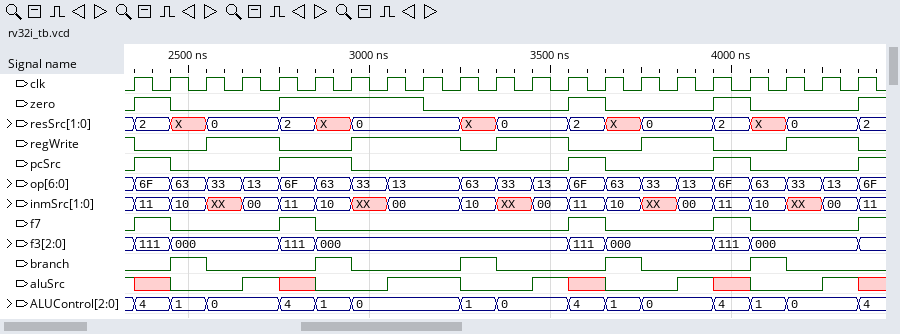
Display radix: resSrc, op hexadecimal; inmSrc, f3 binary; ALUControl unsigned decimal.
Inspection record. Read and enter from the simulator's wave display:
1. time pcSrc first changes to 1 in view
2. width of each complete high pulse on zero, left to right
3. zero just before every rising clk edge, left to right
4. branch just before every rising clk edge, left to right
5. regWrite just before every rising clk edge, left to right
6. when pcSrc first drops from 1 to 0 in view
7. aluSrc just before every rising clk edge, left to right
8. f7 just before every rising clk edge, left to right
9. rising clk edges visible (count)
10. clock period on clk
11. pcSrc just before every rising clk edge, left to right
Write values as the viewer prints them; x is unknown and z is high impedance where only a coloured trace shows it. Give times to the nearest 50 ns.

2350 ns
100 ns, 400 ns, 100 ns, 100 ns
0 1 0 0 0 1 1 1 1 0 0 0 0 1 0 0 0 1 0 0 0
0 0 1 0 0 0 1 0 0 0 1 0 0 0 1 0 0 0 1 0 0
1 0 0 1 1 0 0 1 1 1 0 1 1 0 0 1 1 0 0 1 1
2450 ns
1 x 0 0 1 x 0 0 1 1 0 0 1 x 0 0 1 x 0 0 1
0 1 0 0 0 1 0 0 0 0 0 0 0 1 0 0 0 1 0 0 0
21
100 ns
0 1 0 0 0 1 1 0 0 0 0 0 0 1 0 0 0 1 0 0 0
